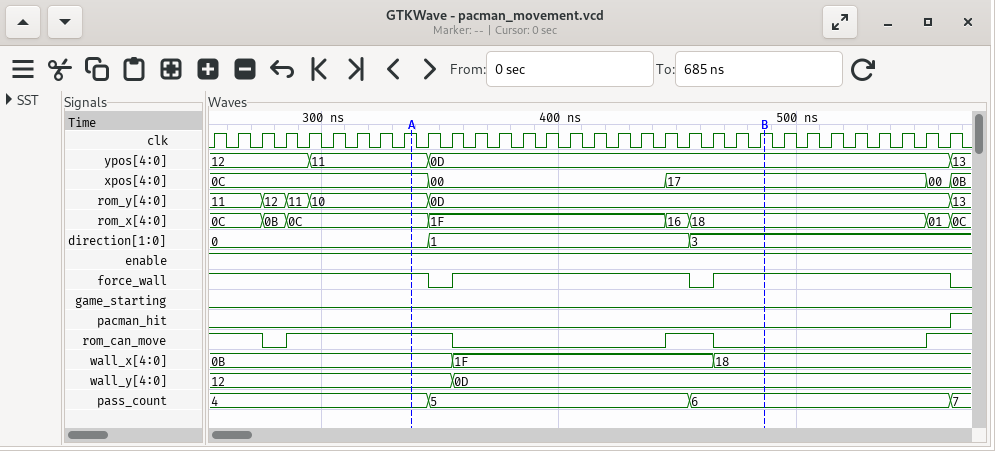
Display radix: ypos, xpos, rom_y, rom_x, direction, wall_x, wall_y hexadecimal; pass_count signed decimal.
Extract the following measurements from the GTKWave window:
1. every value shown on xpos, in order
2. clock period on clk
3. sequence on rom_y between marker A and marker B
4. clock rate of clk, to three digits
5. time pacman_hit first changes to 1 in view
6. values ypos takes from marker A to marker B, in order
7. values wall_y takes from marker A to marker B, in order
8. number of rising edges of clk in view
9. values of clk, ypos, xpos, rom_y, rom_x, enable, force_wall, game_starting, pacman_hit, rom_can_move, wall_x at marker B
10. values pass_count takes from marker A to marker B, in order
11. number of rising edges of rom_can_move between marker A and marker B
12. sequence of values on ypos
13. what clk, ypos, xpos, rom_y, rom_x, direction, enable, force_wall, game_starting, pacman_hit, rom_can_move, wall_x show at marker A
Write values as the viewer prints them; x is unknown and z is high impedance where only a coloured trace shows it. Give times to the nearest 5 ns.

0C, 00, 17, 00, 0B
10 ns
10, 0D
100 MHz
565 ns
11, 0D
12, 0D
32
clk=1, ypos=0D, xpos=17, rom_y=0D, rom_x=18, enable=1, force_wall=1, game_starting=0, pacman_hit=0, rom_can_move=0, wall_x=18
4, 5, 6
1
12, 11, 0D, 13
clk=1, ypos=11, xpos=0C, rom_y=10, rom_x=0C, direction=0, enable=1, force_wall=1, game_starting=0, pacman_hit=0, rom_can_move=1, wall_x=0B
